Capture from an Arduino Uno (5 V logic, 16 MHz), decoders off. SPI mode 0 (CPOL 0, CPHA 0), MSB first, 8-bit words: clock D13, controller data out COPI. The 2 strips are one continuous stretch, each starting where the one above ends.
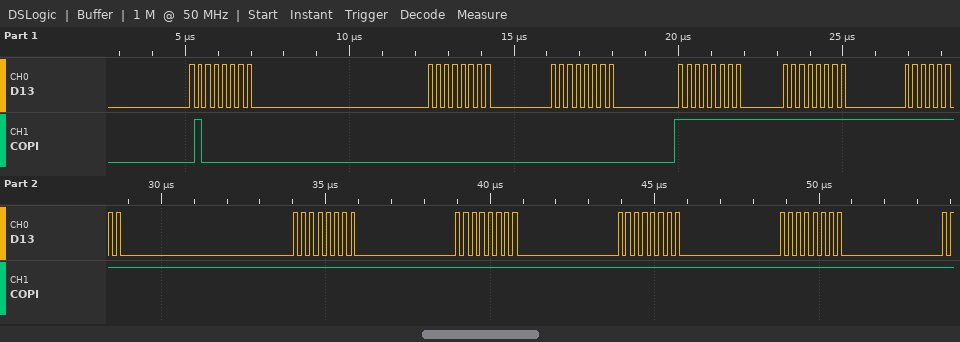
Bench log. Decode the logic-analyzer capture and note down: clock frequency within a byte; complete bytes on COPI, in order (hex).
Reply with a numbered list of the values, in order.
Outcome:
1. 4 MHz
2. 0x40 0x00 0x00 0xFF 0xFF 0xFF 0xFF 0xFF 0xFF 0xFF
